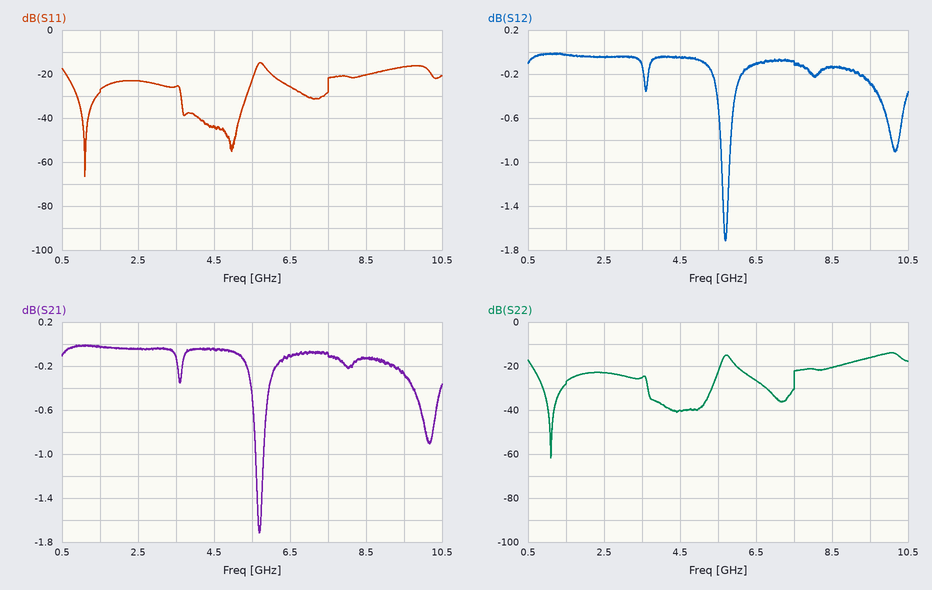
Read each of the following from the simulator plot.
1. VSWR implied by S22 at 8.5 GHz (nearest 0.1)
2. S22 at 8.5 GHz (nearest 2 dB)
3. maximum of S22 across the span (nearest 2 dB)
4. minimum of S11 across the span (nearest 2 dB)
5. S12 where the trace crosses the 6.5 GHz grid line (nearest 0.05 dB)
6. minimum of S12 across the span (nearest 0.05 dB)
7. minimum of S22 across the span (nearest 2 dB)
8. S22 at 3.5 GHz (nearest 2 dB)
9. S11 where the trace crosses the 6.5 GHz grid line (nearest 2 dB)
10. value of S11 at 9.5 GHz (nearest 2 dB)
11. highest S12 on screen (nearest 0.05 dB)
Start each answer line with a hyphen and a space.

- 1.2
- -20 dB
- -14 dB
- -66 dB
- -0.10 dB
- -1.70 dB
- -62 dB
- -26 dB
- -26 dB
- -16 dB
- 0.00 dB
